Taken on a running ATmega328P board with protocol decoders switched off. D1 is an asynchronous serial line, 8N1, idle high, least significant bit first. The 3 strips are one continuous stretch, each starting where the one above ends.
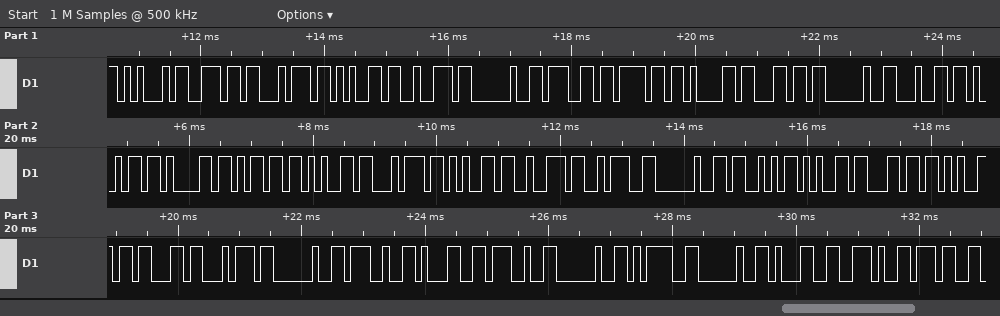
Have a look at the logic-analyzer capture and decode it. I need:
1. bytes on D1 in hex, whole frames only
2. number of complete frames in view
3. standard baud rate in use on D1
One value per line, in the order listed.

45 6E 74 65 72 20 67 6F 61 6C 20 64 69 61 6D 65 74 65 72 3A 20 53 65 6C 65 63 74 20 27 31 27 20 3D 20 31 2E 37
37
9600 baud
